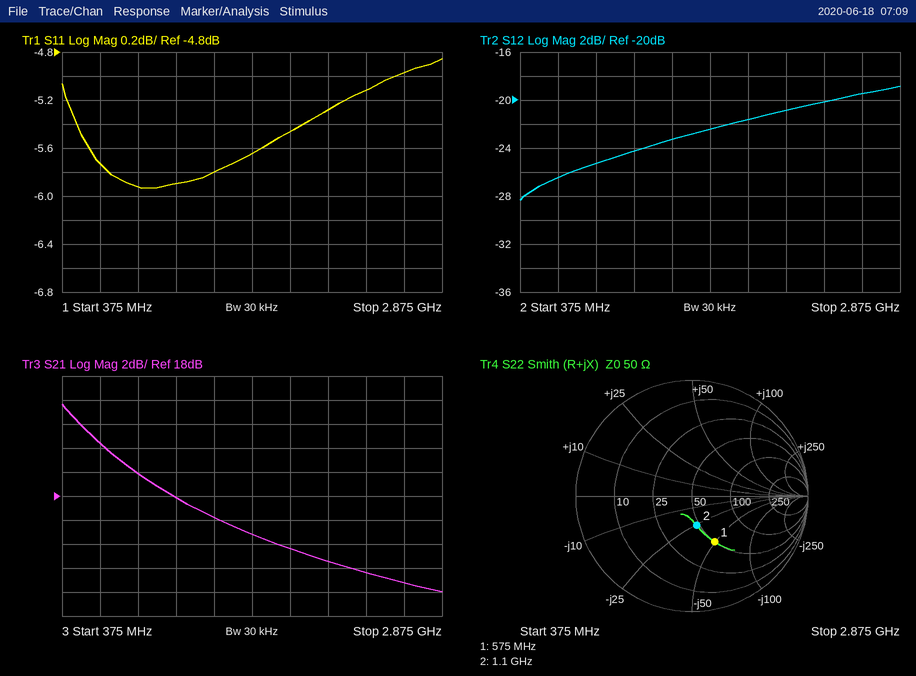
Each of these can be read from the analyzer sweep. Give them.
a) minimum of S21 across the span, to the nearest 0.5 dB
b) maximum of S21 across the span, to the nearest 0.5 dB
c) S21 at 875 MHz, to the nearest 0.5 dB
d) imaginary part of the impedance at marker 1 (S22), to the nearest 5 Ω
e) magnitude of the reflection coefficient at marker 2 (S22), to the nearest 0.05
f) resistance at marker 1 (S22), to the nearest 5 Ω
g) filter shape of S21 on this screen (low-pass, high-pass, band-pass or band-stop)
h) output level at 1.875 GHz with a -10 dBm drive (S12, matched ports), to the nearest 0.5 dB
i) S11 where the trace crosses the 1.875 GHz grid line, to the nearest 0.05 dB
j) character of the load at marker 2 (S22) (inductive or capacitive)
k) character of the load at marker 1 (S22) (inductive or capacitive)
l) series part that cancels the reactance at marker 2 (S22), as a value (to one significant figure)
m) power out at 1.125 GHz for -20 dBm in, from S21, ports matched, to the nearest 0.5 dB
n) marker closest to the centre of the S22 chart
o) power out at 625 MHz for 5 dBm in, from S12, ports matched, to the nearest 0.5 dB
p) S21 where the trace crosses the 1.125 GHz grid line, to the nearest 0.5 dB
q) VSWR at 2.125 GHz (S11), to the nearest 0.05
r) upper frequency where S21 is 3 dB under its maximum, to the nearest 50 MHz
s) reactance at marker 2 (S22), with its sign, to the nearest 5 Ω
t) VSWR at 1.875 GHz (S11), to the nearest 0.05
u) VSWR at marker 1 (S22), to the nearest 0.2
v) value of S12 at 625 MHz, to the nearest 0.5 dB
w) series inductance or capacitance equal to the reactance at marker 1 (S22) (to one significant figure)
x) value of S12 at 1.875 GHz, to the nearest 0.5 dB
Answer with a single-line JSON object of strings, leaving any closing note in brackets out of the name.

{"minimum of S21 across the span, to the nearest 0.5 dB": "10.0 dB", "maximum of S21 across the span, to the nearest 0.5 dB": "25.5 dB", "S21 at 875 MHz, to the nearest 0.5 dB": "20.0 dB", "imaginary part of the impedance at marker 1 (S22), to the nearest 5 Ω": "-50 Ω", "magnitude of the reflection coefficient at marker 2 (S22), to the nearest 0.05": "0.25", "resistance at marker 1 (S22), to the nearest 5 Ω": "50 Ω", "filter shape of S21 on this screen": "low-pass", "output level at 1.875 GHz with a -10 dBm drive (S12, matched ports), to the nearest 0.5 dB": "-31.5 dBm", "S11 where the trace crosses the 1.875 GHz grid line, to the nearest 0.05 dB": "-5.45 dB", "character of the load at marker 2 (S22)": "capacitive", "character of the load at marker 1 (S22)": "capacitive", "series part that cancels the reactance at marker 2 (S22), as a value": "4 nH", "power out at 1.125 GHz for -20 dBm in, from S21, ports matched, to the nearest 0.5 dB": "-2.0 dBm", "marker closest to the centre of the S22 chart": "marker 2", "power out at 625 MHz for 5 dBm in, from S12, ports matched, to the nearest 0.5 dB": "-21.5 dBm", "S21 where the trace crosses the 1.125 GHz grid line, to the nearest 0.5 dB": "18.0 dB", "VSWR at 2.125 GHz (S11), to the nearest 0.05": "3.40", "upper frequency where S21 is 3 dB under its maximum, to the nearest 50 MHz": "600 MHz", "reactance at marker 2 (S22), with its sign, to the nearest 5 Ω": "-25 Ω", "VSWR at 1.875 GHz (S11), to the nearest 0.05": "3.30", "VSWR at marker 1 (S22), to the nearest 0.2": "2.6", "value of S12 at 625 MHz, to the nearest 0.5 dB": "-26.5 dB", "series inductance or capacitance equal to the reactance at marker 1 (S22)": "6 pF", "value of S12 at 1.875 GHz, to the nearest 0.5 dB": "-21.5 dB"}
